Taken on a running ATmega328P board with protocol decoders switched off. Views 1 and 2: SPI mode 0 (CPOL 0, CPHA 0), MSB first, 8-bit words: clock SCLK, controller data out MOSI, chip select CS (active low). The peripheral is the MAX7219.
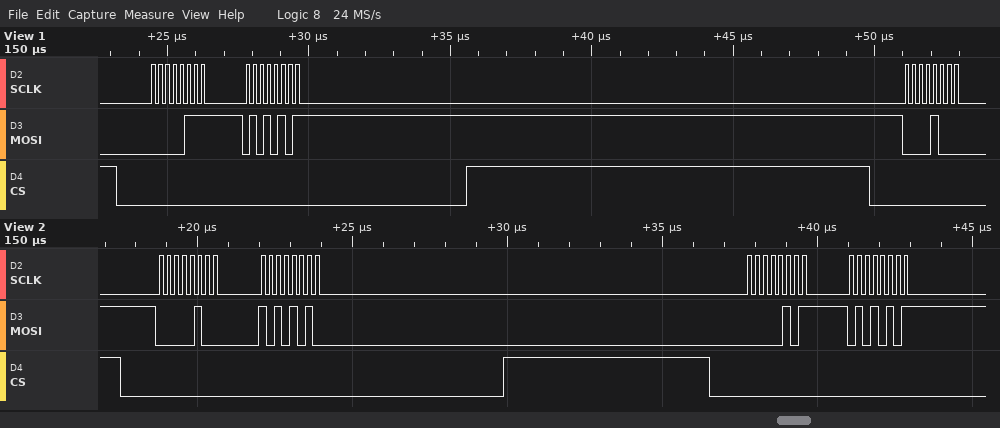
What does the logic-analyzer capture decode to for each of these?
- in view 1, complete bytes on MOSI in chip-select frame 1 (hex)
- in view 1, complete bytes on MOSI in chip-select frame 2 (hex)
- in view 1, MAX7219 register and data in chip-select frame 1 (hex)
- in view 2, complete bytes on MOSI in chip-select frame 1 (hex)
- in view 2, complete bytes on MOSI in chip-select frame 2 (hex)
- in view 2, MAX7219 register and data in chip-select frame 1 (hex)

07 55
08
register 0x7, data 0x55
04 AA
05 55
register 0x4, data 0xAA
